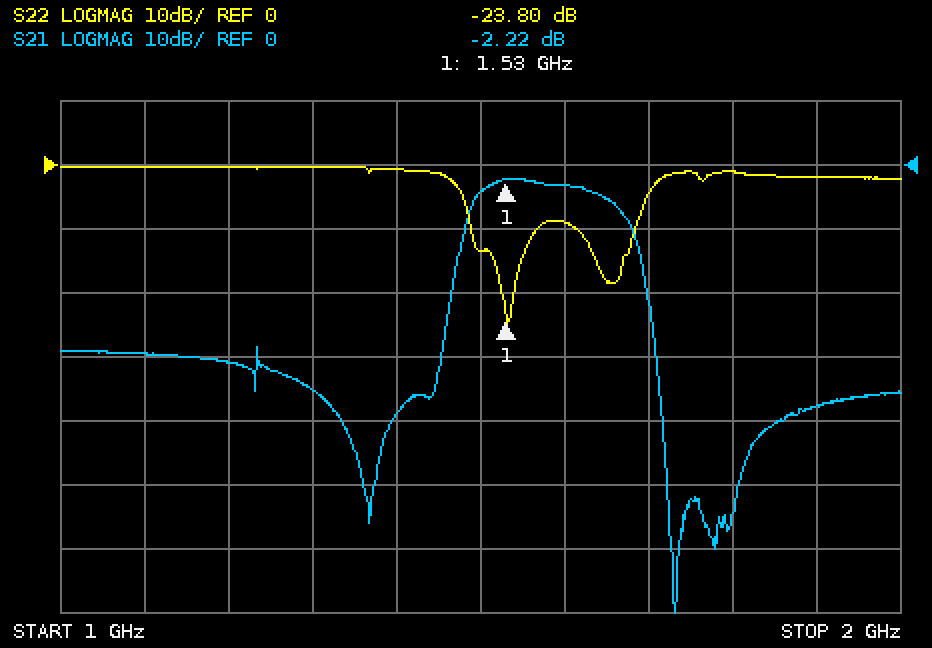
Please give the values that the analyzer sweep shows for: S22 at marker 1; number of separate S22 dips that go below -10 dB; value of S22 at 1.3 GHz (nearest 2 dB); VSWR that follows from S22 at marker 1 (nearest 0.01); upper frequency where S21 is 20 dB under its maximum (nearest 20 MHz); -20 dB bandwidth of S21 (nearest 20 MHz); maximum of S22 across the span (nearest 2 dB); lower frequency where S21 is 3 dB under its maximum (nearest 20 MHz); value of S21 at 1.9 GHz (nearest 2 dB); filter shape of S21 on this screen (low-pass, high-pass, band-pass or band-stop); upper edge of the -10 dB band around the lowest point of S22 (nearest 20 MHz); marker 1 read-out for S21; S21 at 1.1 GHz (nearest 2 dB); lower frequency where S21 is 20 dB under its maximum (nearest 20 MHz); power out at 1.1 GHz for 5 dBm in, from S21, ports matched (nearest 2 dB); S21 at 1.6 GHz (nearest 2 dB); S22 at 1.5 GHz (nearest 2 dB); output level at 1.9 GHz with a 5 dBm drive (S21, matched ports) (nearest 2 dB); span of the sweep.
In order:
-23.80 dB
2
0 dB
1.14
1.70 GHz
240 MHz
0 dB
1.50 GHz
-38 dB
band-pass
1.56 GHz
-2.22 dB
-30 dB
1.46 GHz
-24 dBm
-4 dB
-14 dB
-32 dBm
1 GHz
